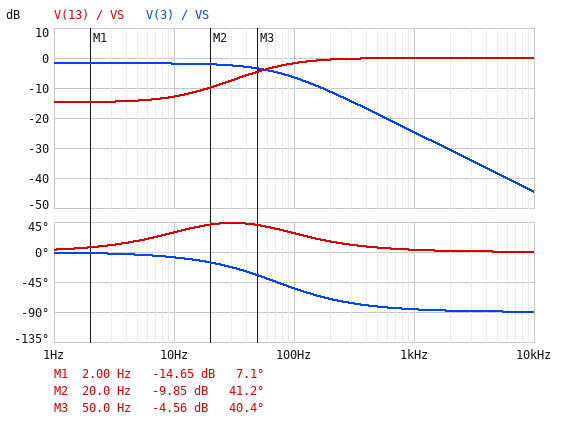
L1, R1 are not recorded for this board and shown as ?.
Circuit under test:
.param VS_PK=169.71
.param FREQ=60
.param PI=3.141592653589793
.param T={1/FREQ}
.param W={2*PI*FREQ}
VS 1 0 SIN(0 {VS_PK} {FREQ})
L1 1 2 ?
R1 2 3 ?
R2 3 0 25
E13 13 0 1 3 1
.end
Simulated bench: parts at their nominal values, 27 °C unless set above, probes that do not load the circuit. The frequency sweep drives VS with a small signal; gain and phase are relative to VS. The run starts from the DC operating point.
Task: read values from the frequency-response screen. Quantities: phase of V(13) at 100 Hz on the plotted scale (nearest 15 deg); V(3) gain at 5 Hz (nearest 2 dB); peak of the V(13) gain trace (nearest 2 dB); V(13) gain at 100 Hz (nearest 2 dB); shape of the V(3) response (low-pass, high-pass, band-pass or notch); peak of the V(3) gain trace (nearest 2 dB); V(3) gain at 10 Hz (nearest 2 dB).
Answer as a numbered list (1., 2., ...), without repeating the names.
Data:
1. 30 deg
2. -2 dB
3. 0 dB
4. -2 dB
5. low-pass
6. -2 dB
7. -2 dB
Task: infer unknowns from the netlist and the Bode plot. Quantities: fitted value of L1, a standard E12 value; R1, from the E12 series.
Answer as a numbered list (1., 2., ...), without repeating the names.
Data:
1. 68 mH
2. 5.6 Ω
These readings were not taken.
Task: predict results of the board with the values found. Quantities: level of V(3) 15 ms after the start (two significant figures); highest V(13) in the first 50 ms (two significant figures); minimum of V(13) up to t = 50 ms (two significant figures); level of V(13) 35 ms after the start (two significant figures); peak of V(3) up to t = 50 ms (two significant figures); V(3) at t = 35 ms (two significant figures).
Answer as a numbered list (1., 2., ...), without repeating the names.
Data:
1. -100 V
2. 110 V
3. -110 V
4. 110 V
5. 110 V
6. -7.3 V
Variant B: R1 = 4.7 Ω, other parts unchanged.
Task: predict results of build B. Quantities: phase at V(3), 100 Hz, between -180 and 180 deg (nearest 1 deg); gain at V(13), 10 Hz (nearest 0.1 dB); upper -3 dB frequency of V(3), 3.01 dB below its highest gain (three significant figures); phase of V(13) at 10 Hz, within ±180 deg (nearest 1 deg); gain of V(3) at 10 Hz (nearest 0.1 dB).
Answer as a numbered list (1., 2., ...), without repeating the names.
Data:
1. -55 deg
2. -13.5 dB
3. 69.5 Hz
4. 34 deg
5. -1.6 dB
